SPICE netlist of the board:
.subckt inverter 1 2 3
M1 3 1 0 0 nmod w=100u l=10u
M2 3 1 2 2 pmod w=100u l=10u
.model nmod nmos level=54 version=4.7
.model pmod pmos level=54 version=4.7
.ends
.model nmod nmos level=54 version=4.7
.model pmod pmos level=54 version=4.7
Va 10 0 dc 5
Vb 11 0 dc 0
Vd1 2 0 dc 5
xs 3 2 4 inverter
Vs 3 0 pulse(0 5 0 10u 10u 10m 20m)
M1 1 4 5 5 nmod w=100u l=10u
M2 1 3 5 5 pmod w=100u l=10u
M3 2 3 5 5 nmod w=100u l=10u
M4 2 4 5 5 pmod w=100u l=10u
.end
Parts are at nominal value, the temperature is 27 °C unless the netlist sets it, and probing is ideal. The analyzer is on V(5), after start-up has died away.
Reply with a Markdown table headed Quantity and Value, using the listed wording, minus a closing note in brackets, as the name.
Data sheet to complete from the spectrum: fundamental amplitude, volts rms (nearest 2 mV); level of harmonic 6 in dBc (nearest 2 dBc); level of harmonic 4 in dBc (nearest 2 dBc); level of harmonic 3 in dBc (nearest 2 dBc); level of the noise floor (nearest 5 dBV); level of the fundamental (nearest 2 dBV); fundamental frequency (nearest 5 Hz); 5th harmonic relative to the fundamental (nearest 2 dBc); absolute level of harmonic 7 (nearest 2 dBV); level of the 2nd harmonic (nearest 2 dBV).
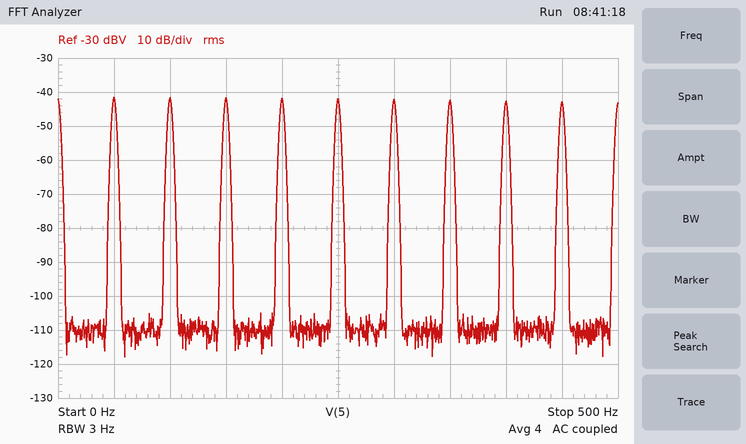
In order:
| Quantity | Value |
|---|---|
| fundamental amplitude, volts rms | 8 mV |
| level of harmonic 6 in dBc | 0 dBc |
| level of harmonic 4 in dBc | 0 dBc |
| level of harmonic 3 in dBc | 0 dBc |
| level of the noise floor | -110 dBV |
| level of the fundamental | -42 dBV |
| fundamental frequency | 50 Hz |
| 5th harmonic relative to the fundamental | 0 dBc |
| absolute level of harmonic 7 | -42 dBV |
| level of the 2nd harmonic | -42 dBV |
